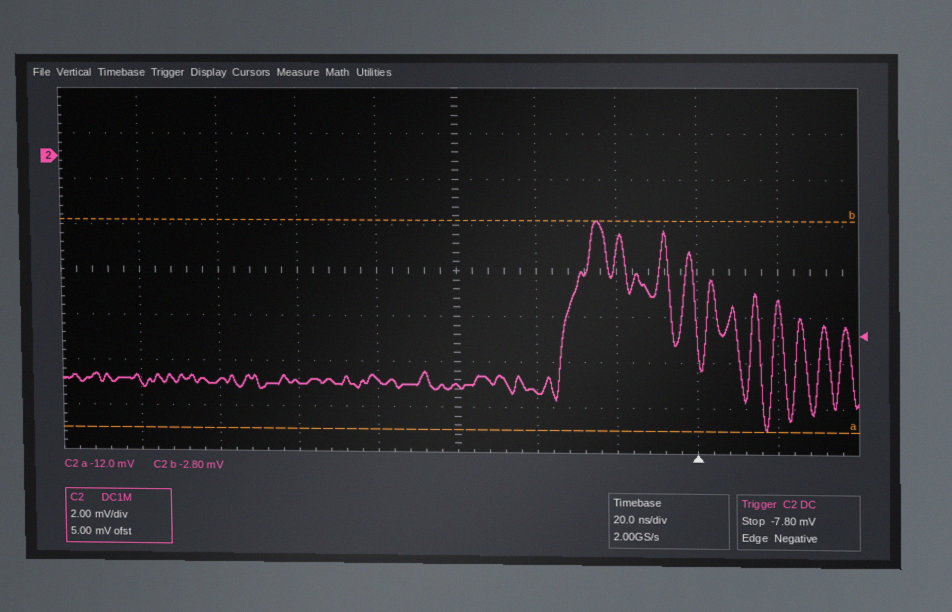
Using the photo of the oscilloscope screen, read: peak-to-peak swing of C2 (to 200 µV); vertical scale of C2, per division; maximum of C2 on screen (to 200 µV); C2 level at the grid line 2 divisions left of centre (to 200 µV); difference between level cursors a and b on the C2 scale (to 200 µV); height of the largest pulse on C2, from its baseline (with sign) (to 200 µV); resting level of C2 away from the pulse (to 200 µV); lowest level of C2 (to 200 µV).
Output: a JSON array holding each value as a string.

["9.2 mV", "2 mV", "-2.8 mV", "-10.0 mV", "9.2 mV", "+7.0 mV", "-9.8 mV", "-12.0 mV"]
